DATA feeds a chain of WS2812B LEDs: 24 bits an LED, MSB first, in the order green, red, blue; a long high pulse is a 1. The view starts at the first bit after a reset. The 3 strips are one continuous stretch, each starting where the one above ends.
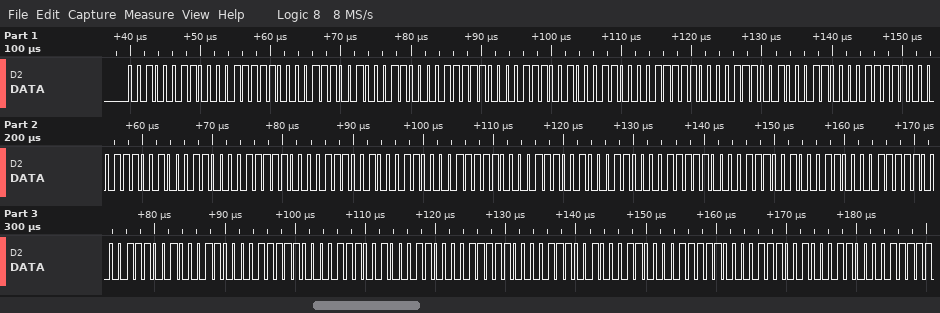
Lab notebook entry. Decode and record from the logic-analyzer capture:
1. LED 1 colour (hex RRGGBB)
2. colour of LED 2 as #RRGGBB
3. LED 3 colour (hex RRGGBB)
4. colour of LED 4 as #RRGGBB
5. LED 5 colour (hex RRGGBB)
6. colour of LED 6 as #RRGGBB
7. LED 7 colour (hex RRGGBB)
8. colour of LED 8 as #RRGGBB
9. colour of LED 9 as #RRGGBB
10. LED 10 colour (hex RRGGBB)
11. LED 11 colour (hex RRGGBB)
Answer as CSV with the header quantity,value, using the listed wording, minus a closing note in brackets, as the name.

quantity,value
LED 1 colour,#0F2387
colour of LED 2 as #RRGGBB,#0F2387
LED 3 colour,#0F2387
colour of LED 4 as #RRGGBB,#0F2387
LED 5 colour,#0F2387
colour of LED 6 as #RRGGBB,#0F2387
LED 7 colour,#0F2387
colour of LED 8 as #RRGGBB,#0F2387
colour of LED 9 as #RRGGBB,#0F2387
LED 10 colour,#0F2387
LED 11 colour,#0F2387
